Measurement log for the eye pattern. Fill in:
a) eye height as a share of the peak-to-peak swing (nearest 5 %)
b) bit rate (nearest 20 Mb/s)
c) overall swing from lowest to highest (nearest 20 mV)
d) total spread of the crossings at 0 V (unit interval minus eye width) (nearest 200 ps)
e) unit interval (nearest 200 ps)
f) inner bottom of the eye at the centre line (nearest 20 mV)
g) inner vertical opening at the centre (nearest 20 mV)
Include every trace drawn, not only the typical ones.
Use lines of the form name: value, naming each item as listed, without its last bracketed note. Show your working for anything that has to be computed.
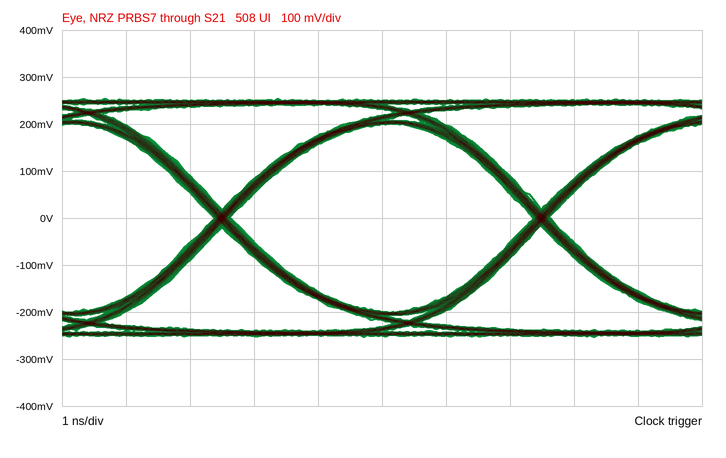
eye height as a share of the peak-to-peak swing: 400 mV / 500 mV ≈ 80 %
bit rate: 200 Mb/s
overall swing from lowest to highest: 500 mV
total spread of the crossings at 0 V (unit interval minus eye width): 200 ps
unit interval: 5.0 ns
inner bottom of the eye at the centre line: -200 mV
inner vertical opening at the centre: 400 mV
